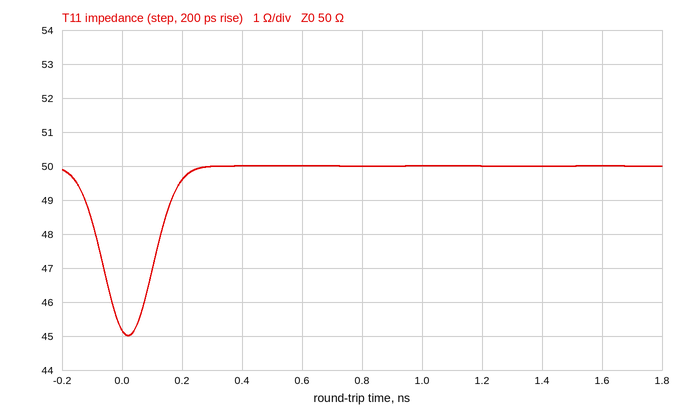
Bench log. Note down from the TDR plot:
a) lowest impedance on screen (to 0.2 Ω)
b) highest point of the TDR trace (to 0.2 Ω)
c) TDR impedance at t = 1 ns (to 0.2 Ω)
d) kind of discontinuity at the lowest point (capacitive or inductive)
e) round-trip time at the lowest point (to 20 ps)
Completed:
45.0 Ω
50.0 Ω
50.0 Ω
capacitive
20 ps
